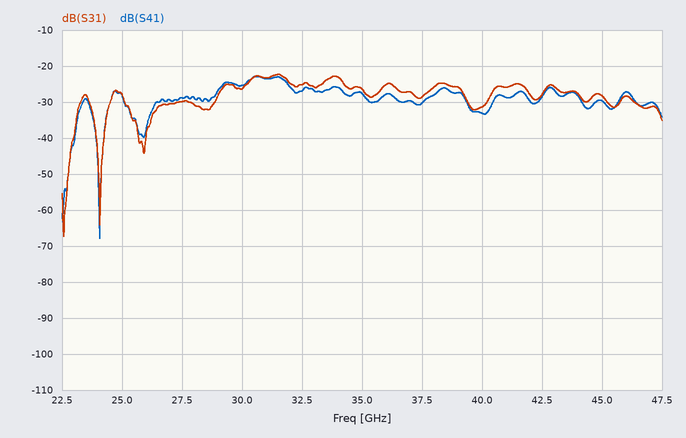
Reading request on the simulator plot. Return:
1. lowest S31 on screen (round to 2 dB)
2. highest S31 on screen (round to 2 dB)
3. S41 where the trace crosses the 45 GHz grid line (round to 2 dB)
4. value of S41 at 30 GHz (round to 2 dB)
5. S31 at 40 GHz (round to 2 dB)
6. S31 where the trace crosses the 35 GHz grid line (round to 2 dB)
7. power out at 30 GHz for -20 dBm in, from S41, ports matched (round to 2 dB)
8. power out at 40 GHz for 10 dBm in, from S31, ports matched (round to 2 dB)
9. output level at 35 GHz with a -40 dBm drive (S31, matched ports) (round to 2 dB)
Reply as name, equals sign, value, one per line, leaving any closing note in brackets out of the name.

lowest S31 on screen = -68 dB
highest S31 on screen = -22 dB
S41 where the trace crosses the 45 GHz grid line = -30 dB
value of S41 at 30 GHz = -26 dB
S31 at 40 GHz = -32 dB
S31 where the trace crosses the 35 GHz grid line = -26 dB
power out at 30 GHz for -20 dBm in, from S41, ports matched = -46 dBm
power out at 40 GHz for 10 dBm in, from S31, ports matched = -22 dBm
output level at 35 GHz with a -40 dBm drive (S31, matched ports) = -66 dBm
